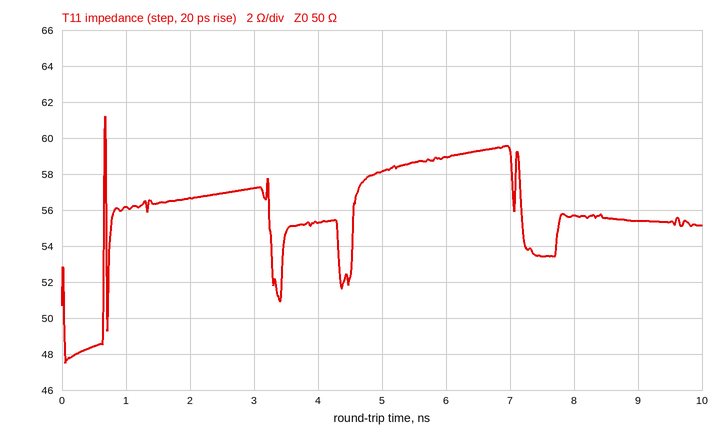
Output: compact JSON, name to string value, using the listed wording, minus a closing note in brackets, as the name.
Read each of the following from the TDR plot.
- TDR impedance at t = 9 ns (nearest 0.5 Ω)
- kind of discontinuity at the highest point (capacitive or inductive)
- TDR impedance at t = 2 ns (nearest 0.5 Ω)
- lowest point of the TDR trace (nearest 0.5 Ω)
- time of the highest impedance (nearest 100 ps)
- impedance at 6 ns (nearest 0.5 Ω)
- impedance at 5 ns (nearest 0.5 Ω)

{"TDR impedance at t = 9 ns": "55.5 Ω", "kind of discontinuity at the highest point": "inductive", "TDR impedance at t = 2 ns": "56.5 Ω", "lowest point of the TDR trace": "47.5 Ω", "time of the highest impedance": "700 ps", "impedance at 6 ns": "59.0 Ω", "impedance at 5 ns": "58.0 Ω"}
